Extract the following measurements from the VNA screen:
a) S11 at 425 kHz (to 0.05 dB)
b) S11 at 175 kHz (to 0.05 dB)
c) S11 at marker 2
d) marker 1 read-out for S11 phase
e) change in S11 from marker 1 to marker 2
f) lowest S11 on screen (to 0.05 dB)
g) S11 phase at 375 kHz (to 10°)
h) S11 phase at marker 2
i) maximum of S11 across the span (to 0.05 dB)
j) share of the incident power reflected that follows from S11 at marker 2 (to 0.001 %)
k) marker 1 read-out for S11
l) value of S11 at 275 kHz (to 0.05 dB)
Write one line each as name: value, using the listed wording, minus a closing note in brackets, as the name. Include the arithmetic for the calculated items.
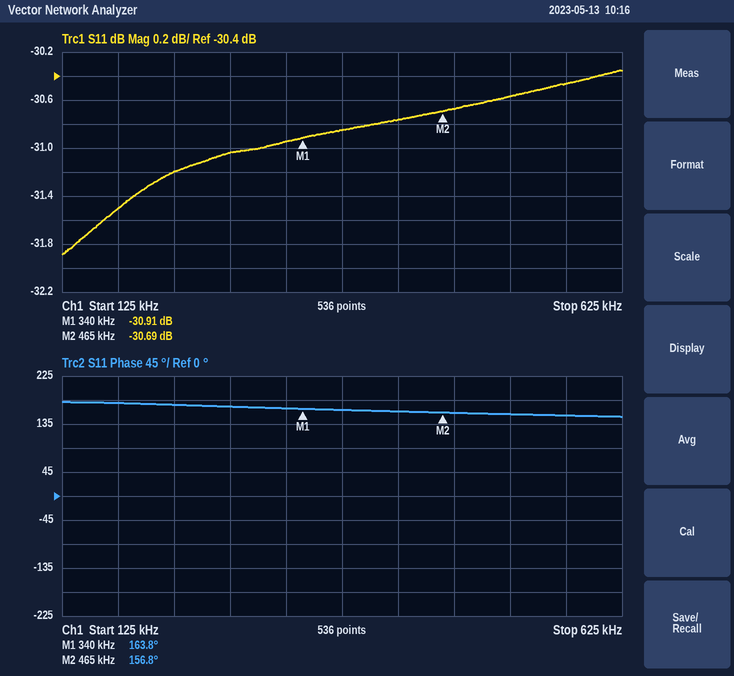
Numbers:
S11 at 425 kHz: -30.75 dB
S11 at 175 kHz: -31.50 dB
S11 at marker 2: -30.69 dB
marker 1 read-out for S11 phase: 163.8°
change in S11 from marker 1 to marker 2: -30.69 − (-30.91) = 0.22 dB
lowest S11 on screen: -31.90 dB
S11 phase at 375 kHz: 160°
S11 phase at marker 2: 156.8°
maximum of S11 across the span: -30.35 dB
share of the incident power reflected that follows from S11 at marker 2: 10^(-30.69/10) ≈ 0.085 %
marker 1 read-out for S11: -30.91 dB
value of S11 at 275 kHz: -31.05 dB
